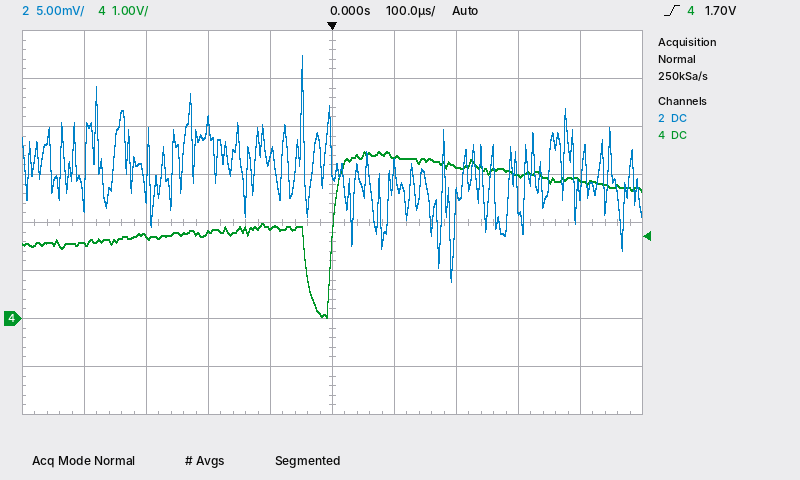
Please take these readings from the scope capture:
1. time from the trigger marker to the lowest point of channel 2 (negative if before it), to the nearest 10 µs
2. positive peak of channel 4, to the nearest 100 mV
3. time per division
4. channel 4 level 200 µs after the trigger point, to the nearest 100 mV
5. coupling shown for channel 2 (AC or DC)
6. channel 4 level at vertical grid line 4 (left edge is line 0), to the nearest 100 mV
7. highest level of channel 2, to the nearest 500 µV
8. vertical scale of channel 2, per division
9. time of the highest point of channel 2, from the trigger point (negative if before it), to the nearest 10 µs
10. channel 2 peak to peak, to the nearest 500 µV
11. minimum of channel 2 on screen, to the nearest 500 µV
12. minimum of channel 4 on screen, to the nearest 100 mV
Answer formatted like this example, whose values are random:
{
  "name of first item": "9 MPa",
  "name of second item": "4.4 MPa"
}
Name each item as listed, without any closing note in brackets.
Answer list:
{
  "time from the trigger marker to the lowest point of channel 2 (negative if before it), to the nearest 10 µs": "+190 µs",
  "positive peak of channel 4, to the nearest 100 mV": "3.5 V",
  "time per division": "100 µs",
  "channel 4 level 200 µs after the trigger point, to the nearest 100 mV": "3.2 V",
  "coupling shown for channel 2": "DC",
  "channel 4 level at vertical grid line 4 (left edge is line 0), to the nearest 100 mV": "1.9 V",
  "highest level of channel 2, to the nearest 500 µV": "27.5 mV",
  "vertical scale of channel 2, per division": "5 mV",
  "time of the highest point of channel 2, from the trigger point (negative if before it), to the nearest 10 µs": "-50 µs",
  "channel 2 peak to peak, to the nearest 500 µV": "23.5 mV",
  "minimum of channel 2 on screen, to the nearest 500 µV": "4.0 mV",
  "minimum of channel 4 on screen, to the nearest 100 mV": "0.0 V"
}
